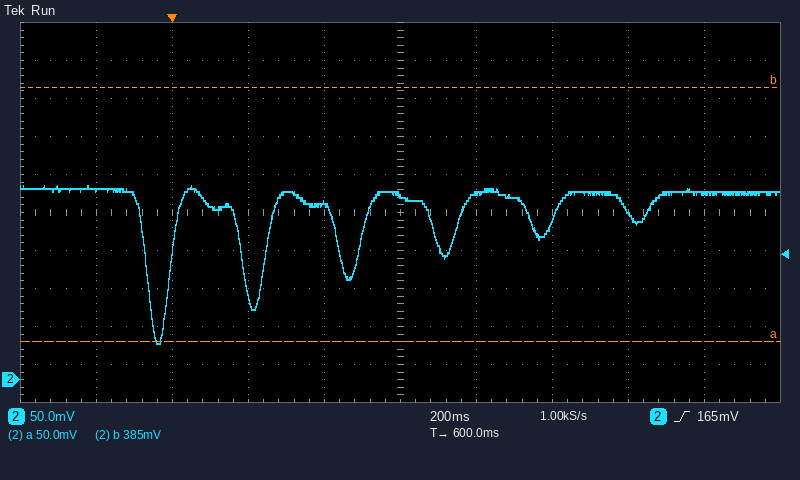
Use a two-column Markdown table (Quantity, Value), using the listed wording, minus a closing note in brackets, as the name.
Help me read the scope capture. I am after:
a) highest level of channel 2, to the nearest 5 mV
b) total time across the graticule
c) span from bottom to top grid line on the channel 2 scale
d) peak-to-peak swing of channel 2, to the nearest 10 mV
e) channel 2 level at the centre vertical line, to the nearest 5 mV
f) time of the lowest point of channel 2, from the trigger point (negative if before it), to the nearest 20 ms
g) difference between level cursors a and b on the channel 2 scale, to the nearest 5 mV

| Quantity | Value |
|---|---|
| highest level of channel 2, to the nearest 5 mV | 255 mV |
| total time across the graticule | 2 s |
| span from bottom to top grid line on the channel 2 scale | 500 mV |
| peak-to-peak swing of channel 2, to the nearest 10 mV | 210 mV |
| channel 2 level at the centre vertical line, to the nearest 5 mV | 245 mV |
| time of the lowest point of channel 2, from the trigger point (negative if before it), to the nearest 20 ms | -40 ms |
| difference between level cursors a and b on the channel 2 scale, to the nearest 5 mV | 335 mV |
